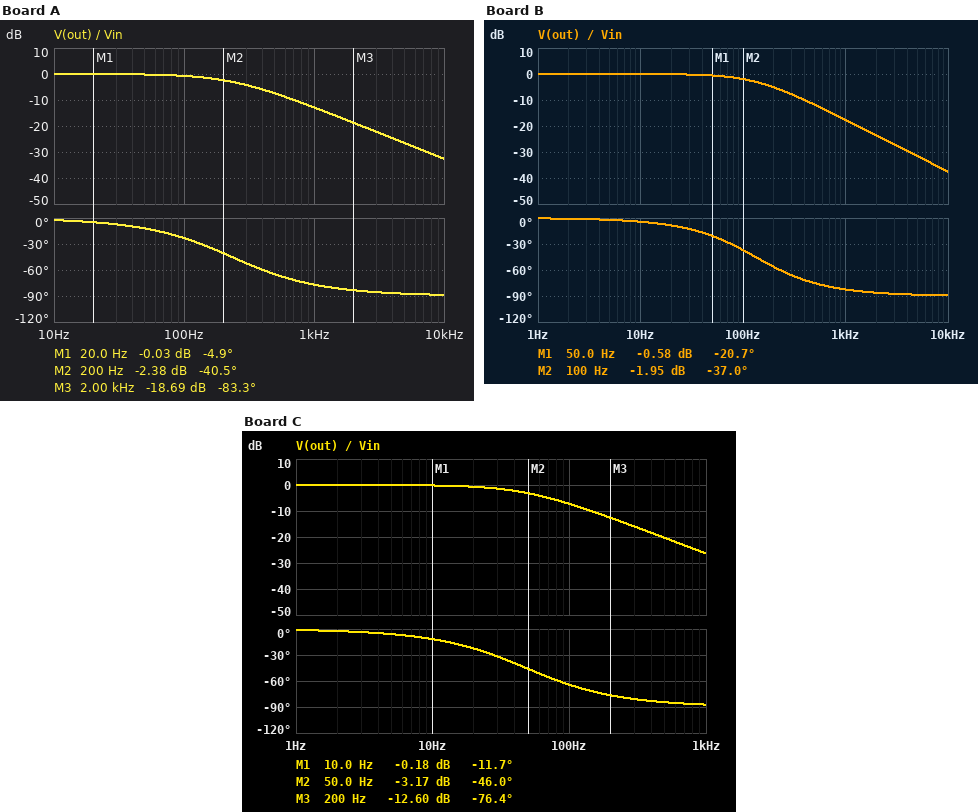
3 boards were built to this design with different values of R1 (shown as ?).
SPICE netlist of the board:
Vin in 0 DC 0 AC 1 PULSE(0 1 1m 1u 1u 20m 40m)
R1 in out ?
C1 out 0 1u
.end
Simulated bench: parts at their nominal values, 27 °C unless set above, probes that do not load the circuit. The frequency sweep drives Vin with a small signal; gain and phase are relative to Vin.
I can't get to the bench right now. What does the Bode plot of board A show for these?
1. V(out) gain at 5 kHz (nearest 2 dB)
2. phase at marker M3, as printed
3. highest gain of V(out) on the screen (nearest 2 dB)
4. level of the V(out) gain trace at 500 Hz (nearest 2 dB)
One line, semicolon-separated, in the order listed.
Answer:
-26 dB; -83.3 deg; 0 dB; -8 dB
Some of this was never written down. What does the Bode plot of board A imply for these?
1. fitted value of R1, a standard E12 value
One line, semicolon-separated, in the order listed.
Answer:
680 Ω
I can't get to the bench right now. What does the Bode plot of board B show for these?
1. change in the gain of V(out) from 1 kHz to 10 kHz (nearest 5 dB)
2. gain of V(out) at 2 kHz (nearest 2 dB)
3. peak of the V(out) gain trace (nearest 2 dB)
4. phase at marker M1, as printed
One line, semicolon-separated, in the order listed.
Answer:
-20 dB; -24 dB; 0 dB; -20.7 deg
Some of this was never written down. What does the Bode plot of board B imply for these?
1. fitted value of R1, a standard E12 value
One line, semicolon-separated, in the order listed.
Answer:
1.2 kΩ
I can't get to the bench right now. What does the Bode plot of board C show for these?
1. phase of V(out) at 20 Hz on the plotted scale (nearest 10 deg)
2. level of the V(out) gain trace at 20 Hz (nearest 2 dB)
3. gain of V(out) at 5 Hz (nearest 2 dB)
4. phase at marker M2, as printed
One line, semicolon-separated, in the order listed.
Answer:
-20 deg; 0 dB; 0 dB; -46.0 deg
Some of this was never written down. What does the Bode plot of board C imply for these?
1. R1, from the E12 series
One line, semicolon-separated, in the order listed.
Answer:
3.3 kΩ
